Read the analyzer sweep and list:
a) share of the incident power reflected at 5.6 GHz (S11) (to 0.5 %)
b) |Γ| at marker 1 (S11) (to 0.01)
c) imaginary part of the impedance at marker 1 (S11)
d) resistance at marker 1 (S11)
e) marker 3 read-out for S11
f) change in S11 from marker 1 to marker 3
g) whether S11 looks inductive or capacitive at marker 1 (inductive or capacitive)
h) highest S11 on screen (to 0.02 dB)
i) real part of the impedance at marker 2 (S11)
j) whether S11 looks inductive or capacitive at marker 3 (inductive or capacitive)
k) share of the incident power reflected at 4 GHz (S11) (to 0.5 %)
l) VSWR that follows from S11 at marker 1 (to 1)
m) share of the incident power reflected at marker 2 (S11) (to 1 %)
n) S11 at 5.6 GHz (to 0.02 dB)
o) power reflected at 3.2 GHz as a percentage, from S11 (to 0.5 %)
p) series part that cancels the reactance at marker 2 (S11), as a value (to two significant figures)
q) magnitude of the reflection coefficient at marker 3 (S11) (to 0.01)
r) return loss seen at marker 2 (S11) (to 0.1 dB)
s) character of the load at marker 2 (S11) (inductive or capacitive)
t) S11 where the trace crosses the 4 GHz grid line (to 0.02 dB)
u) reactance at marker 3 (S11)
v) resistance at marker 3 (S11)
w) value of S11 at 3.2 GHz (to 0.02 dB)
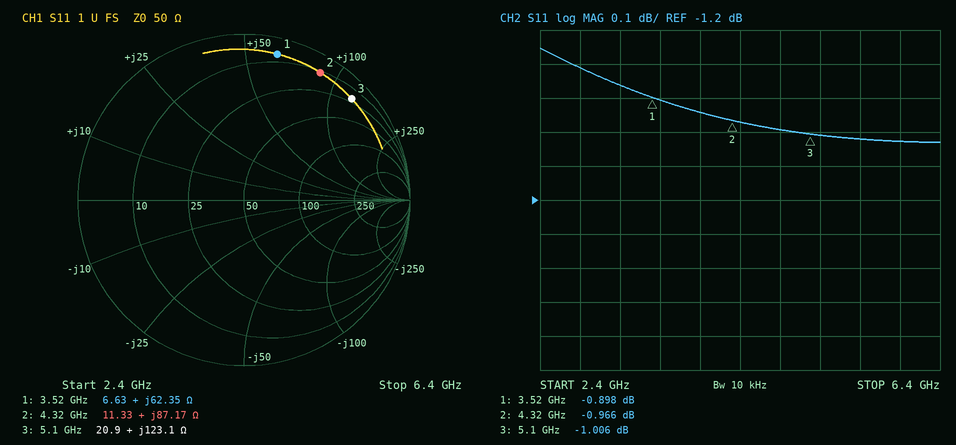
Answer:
79.0 %
0.90
+62.35 Ω
6.63 Ω
-1.006 dB
-0.108 dB
inductive
-0.76 dB
11.33 Ω
inductive
80.5 %
19
80 %
-1.02 dB
82.0 %
420 fF
0.89
1.0 dB
inductive
-0.94 dB
+123.1 Ω
20.9 Ω
-0.86 dB
